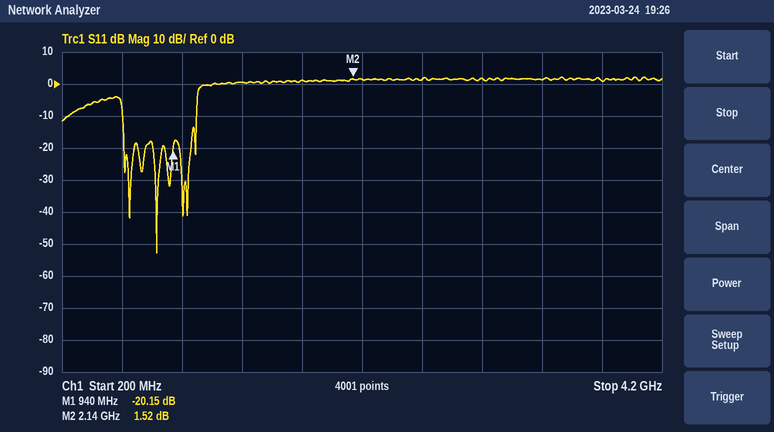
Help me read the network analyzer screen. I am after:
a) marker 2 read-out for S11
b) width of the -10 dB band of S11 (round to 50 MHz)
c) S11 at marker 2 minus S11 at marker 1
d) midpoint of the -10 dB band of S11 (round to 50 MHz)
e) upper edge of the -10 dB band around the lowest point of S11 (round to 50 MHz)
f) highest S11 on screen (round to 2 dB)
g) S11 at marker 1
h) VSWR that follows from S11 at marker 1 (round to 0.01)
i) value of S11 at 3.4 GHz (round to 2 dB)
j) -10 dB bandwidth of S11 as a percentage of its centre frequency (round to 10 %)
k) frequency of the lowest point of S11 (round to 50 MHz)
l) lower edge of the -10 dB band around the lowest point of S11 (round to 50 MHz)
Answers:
1.52 dB
500 MHz
21.67 dB
850 MHz
1.10 GHz
2 dB
-20.15 dB
1.22
2 dB
60 %
850 MHz
600 MHz
